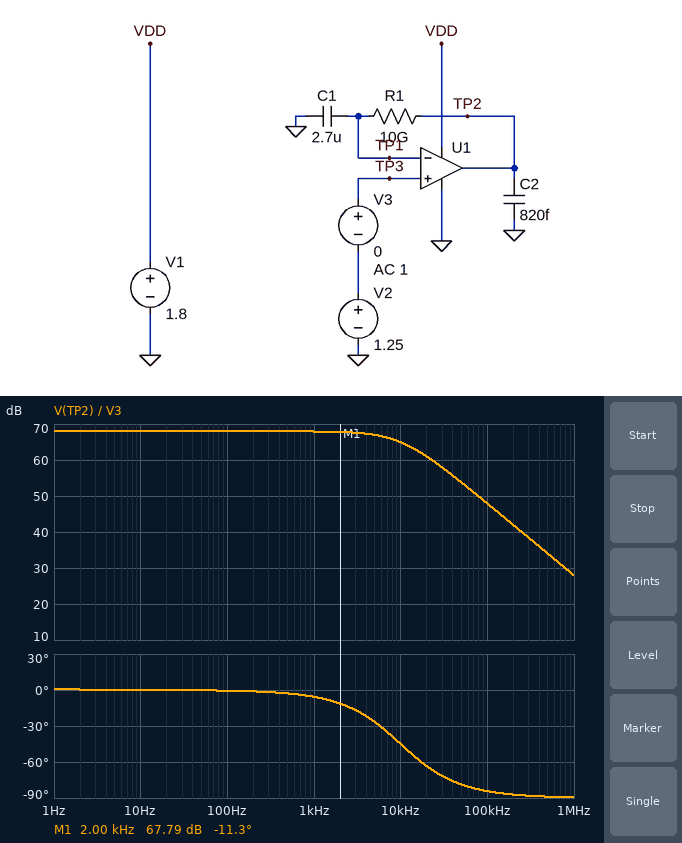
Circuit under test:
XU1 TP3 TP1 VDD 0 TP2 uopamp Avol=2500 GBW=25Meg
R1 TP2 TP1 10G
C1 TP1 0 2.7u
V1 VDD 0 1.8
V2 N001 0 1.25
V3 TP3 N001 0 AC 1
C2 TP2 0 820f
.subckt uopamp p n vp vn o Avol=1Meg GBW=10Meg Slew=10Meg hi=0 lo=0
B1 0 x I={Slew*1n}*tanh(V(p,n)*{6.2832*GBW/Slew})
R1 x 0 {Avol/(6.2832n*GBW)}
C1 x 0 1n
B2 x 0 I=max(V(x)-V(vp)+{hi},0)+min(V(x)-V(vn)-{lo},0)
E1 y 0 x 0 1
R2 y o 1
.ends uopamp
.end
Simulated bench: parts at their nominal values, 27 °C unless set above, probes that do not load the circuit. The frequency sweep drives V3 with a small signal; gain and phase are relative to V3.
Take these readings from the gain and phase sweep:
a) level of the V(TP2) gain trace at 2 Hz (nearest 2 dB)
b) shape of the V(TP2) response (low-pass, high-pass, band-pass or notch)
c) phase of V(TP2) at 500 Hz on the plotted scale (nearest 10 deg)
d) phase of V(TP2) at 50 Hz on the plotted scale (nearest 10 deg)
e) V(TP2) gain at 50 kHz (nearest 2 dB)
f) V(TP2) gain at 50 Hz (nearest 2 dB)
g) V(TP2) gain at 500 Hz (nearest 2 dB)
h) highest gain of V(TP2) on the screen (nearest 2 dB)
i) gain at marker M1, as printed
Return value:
68 dB
low-pass
0 deg
0 deg
54 dB
68 dB
68 dB
68 dB
67.79 dB
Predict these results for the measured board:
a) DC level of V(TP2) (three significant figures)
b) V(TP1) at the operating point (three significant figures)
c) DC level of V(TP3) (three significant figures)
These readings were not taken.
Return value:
1.25 V
1.25 V
1.25 V
